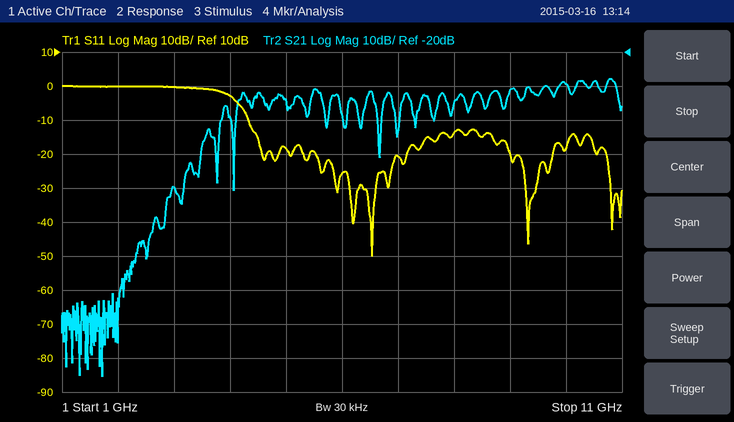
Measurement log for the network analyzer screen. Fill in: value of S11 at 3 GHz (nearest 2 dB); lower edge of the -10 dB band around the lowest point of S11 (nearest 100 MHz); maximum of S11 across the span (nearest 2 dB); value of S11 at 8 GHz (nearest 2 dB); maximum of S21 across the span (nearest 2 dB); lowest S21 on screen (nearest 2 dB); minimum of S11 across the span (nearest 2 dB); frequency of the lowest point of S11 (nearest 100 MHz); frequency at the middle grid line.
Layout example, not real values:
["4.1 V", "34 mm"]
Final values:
["0 dB", "4.3 GHz", "0 dB", "-14 dB", "-28 dB", "-116 dB", "-50 dB", "6.5 GHz", "6 GHz"]
